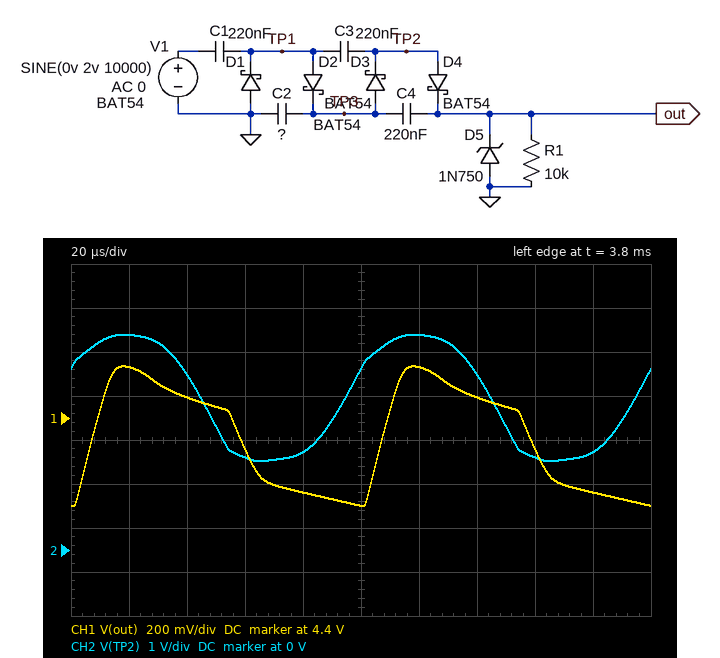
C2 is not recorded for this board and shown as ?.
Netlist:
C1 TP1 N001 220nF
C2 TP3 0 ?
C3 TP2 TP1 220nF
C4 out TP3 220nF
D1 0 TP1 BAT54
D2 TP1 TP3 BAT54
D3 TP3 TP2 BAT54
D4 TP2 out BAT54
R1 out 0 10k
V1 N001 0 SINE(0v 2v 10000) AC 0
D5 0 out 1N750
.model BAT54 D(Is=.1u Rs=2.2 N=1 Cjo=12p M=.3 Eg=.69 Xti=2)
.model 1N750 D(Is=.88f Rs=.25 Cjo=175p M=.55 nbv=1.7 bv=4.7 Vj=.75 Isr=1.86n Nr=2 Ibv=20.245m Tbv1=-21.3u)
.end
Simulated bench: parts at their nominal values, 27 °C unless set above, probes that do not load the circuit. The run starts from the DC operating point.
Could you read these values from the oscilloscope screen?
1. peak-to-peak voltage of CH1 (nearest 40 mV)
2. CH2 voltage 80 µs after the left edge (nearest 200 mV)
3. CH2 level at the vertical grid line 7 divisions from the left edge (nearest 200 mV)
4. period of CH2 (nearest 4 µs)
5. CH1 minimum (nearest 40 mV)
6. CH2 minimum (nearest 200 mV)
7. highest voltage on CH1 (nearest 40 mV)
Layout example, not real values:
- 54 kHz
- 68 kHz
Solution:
- 640 mV
- 2.2 V
- 4.0 V
- 100 µs
- 4.00 V
- 2.0 V
- 4.64 V
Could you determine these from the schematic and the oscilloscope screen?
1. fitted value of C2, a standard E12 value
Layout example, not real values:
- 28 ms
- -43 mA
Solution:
- 330 nF
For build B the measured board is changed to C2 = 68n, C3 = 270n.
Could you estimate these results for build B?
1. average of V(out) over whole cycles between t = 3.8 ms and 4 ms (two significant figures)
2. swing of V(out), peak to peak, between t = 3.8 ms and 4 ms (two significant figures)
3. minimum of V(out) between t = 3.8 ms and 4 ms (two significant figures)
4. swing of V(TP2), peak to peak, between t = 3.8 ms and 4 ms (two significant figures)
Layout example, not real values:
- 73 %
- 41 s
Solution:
- 3.9 V
- 1.5 V
- 3.1 V
- 3.3 V
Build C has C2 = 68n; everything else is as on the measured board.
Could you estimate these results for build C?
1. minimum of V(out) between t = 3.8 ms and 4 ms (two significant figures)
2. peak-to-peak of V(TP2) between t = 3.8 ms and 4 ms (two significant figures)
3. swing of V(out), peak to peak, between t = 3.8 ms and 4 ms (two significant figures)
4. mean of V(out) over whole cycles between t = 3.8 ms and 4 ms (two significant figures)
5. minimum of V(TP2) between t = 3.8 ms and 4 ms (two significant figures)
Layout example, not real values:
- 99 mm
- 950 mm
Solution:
- 3.1 V
- 3.3 V
- 1.5 V
- 3.9 V
- 1.6 V
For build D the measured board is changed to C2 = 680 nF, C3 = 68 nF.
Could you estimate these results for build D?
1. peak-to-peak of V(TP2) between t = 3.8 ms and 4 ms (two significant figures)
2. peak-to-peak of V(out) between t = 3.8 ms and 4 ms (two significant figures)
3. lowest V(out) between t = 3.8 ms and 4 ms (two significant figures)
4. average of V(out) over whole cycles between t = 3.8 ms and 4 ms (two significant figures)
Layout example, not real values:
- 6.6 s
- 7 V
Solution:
- 2.4 V
- 380 mV
- 4.2 V
- 4.4 V
